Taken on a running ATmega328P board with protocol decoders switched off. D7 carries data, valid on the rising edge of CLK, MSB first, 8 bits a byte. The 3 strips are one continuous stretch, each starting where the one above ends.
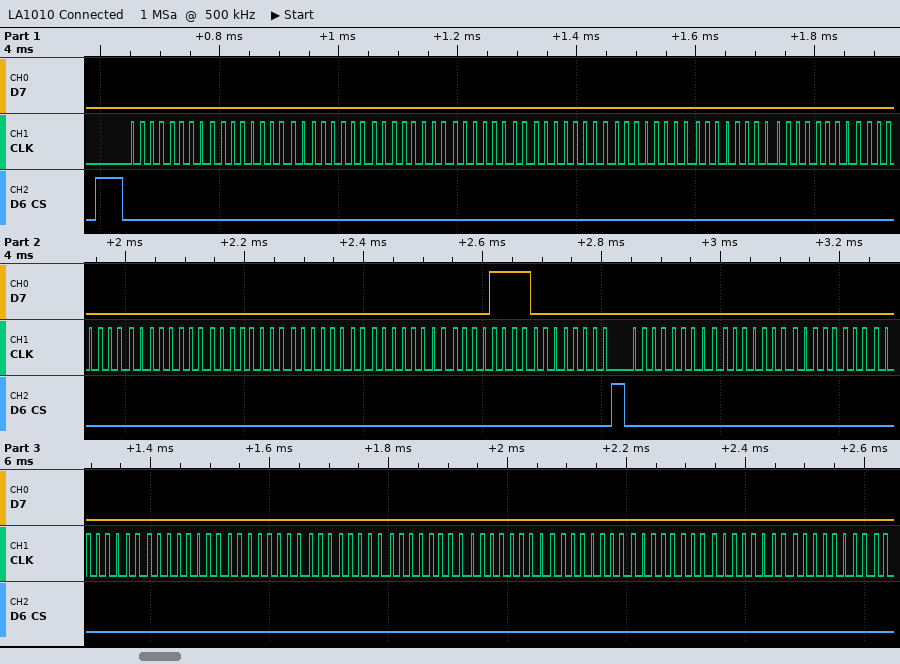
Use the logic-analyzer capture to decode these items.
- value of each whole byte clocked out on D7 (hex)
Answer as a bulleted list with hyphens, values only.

- 00 00 00 00 00 00 00 00 00 00 00 00 00 00 0F 00 00 00 00 00 00 00 00 00 00 00 00 00 00
